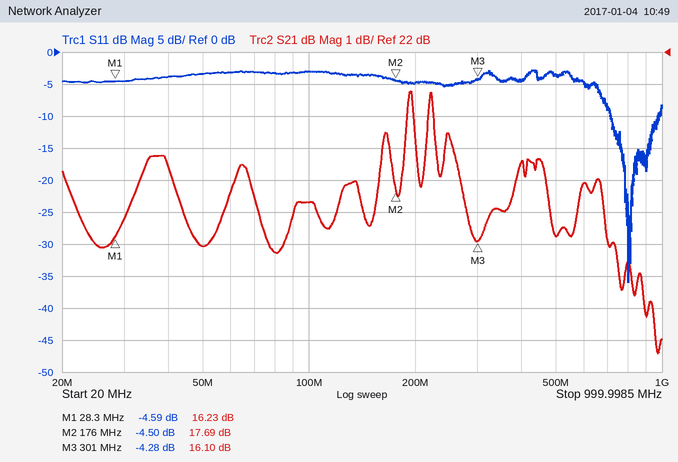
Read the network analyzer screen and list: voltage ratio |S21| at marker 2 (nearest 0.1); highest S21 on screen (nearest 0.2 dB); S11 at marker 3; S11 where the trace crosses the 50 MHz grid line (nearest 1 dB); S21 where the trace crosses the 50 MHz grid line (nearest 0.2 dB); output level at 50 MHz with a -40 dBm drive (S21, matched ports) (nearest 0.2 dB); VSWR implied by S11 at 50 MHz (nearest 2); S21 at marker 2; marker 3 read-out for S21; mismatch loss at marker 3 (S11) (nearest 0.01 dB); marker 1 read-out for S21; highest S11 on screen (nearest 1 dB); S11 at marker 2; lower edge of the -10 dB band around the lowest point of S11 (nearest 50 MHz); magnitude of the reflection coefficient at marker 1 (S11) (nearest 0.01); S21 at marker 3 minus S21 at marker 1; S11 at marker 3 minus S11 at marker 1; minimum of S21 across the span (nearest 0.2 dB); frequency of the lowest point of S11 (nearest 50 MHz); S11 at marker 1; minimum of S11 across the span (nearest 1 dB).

7.7
20.8 dB
-4.28 dB
-3 dB
16.0 dB
-24.0 dBm
6
17.69 dB
16.10 dB
2.03 dB
16.23 dB
-3 dB
-4.50 dB
700 MHz
0.59
-0.13 dB
0.31 dB
12.6 dB
800 MHz
-4.59 dB
-36 dB
